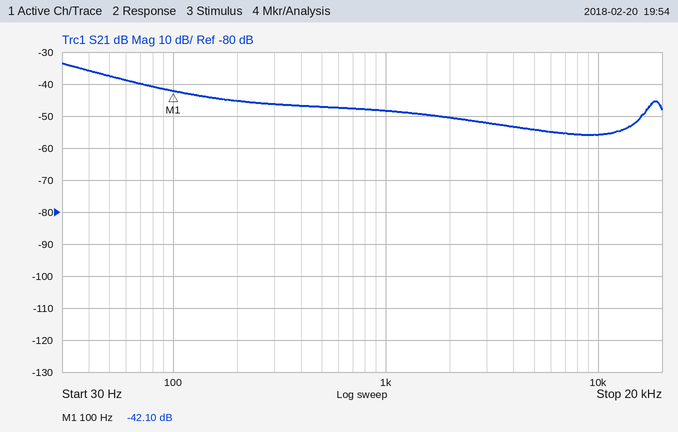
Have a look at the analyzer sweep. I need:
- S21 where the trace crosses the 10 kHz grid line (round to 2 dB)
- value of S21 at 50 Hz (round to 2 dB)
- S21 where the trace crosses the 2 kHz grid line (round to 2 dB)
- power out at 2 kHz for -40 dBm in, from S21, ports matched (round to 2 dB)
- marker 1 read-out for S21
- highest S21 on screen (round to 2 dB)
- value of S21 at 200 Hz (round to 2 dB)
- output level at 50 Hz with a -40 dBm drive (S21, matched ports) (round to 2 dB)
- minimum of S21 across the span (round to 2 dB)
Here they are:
-56 dB
-38 dB
-50 dB
-90 dBm
-42.10 dB
-34 dB
-46 dB
-78 dBm
-56 dB
